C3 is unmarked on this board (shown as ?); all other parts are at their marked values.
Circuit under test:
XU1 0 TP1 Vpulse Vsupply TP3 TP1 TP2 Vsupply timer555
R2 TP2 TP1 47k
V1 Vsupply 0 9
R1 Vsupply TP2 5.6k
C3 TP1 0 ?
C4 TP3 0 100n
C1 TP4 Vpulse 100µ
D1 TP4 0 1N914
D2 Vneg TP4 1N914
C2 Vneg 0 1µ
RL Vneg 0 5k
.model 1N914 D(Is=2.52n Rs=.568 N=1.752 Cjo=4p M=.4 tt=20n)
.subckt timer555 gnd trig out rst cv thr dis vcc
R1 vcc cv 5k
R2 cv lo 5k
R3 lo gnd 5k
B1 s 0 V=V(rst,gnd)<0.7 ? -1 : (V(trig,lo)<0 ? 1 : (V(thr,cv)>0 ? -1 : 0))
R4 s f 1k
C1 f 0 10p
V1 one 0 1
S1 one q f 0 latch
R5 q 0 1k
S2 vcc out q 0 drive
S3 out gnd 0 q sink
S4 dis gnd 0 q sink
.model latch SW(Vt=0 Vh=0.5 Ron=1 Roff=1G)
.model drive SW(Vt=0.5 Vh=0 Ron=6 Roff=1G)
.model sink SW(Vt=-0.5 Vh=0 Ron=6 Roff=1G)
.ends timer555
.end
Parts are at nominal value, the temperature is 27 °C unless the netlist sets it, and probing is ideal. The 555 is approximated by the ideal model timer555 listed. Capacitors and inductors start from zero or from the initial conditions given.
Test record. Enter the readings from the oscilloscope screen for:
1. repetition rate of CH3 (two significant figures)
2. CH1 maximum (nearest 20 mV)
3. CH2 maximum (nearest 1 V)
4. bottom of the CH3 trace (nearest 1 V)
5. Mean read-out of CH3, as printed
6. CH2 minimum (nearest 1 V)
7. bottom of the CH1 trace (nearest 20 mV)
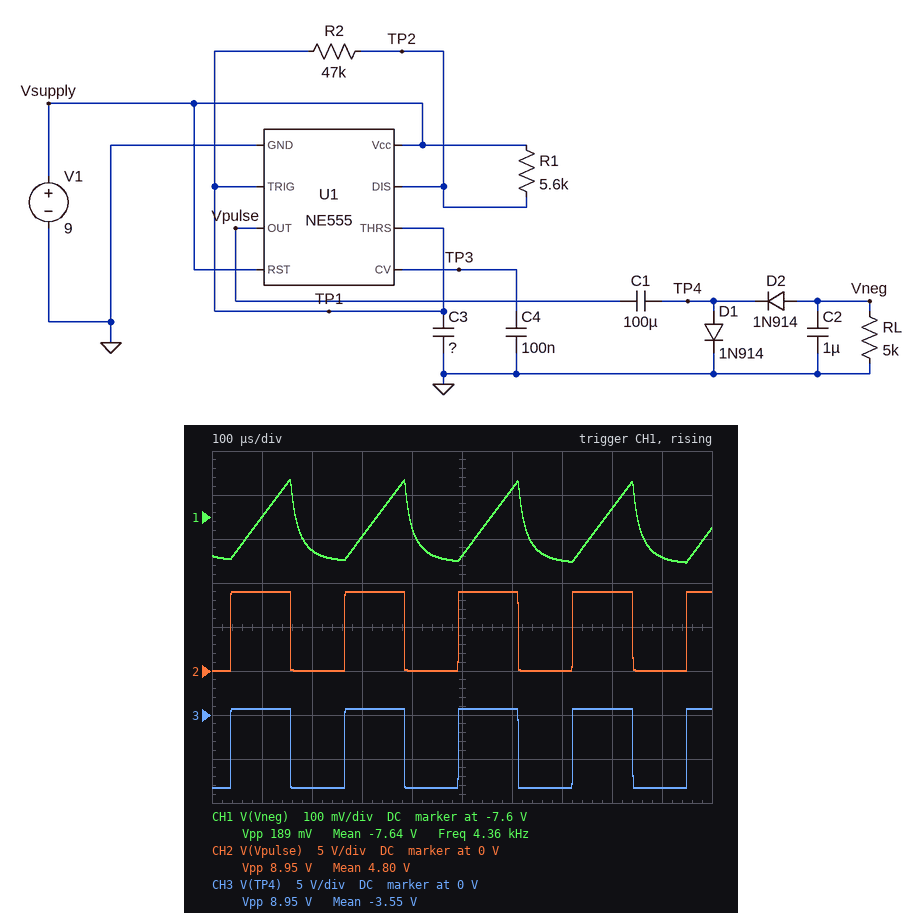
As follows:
4.4 kHz
-7.52 V
9 V
-8 V
-3.55 V
0 V
-7.70 V
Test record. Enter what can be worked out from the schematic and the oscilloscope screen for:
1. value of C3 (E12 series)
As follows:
3.3 nF
